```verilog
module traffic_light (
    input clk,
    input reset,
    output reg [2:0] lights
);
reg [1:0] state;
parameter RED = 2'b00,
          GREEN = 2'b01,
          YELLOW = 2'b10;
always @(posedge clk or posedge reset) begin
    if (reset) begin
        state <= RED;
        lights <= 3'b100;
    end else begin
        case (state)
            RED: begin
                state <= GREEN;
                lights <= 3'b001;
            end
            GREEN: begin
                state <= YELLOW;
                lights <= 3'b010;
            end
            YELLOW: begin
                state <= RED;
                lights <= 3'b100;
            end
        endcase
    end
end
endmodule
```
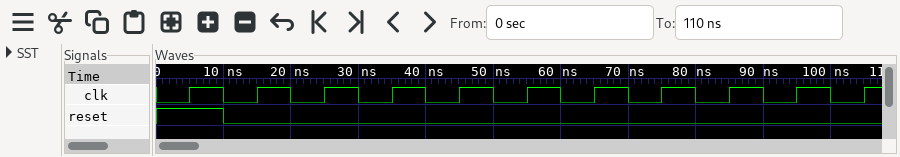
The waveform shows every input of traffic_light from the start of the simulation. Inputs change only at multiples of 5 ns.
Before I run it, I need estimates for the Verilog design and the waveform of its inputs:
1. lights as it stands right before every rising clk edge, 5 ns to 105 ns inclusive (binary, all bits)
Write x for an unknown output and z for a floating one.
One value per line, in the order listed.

100, 100, 001, 010, 100, 001, 010, 100, 001, 010, 100
